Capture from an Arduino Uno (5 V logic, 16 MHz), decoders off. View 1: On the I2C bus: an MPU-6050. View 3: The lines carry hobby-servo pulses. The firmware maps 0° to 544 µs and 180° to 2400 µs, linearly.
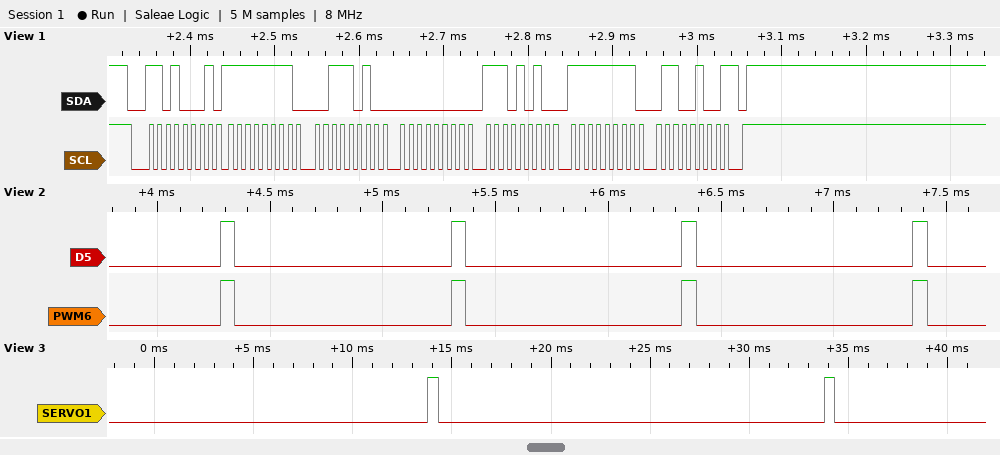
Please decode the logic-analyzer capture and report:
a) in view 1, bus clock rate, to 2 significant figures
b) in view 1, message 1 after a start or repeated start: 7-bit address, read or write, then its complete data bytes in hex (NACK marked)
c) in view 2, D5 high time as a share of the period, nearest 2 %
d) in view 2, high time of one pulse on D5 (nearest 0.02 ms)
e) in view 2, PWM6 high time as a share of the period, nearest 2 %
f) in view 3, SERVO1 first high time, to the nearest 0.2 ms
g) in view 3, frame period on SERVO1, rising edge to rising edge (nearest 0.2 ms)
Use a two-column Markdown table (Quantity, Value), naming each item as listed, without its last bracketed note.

| Quantity | Value |
|---|---|
| in view 1, bus clock rate, to 2 significant figures | 100 kHz |
| in view 1, message 1 after a start or repeated start: 7-bit address, read or write, then its complete data bytes in hex | 0x68 read: FF 3A 00 EA FF 64 NACK |
| in view 2, D5 high time as a share of the period, nearest 2 % | 6 % |
| in view 2, high time of one pulse on D5 | 0.06 ms |
| in view 2, PWM6 high time as a share of the period, nearest 2 % | 6 % |
| in view 3, SERVO1 first high time, to the nearest 0.2 ms | 0.6 ms |
| in view 3, frame period on SERVO1, rising edge to rising edge | 20.0 ms |
